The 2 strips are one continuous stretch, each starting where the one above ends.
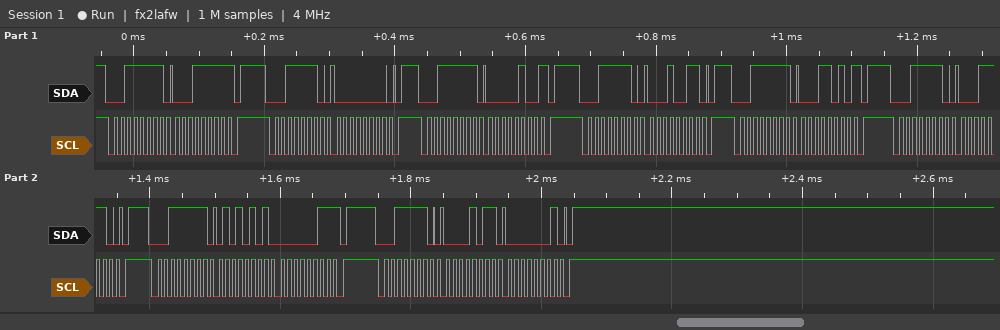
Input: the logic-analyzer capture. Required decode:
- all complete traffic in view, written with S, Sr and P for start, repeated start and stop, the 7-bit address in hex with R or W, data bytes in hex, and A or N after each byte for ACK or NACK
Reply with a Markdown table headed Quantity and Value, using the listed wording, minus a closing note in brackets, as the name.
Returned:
| Quantity | Value |
|---|---|
| all complete traffic in view, written with S, Sr and P for start, repeated start and stop, the 7-bit address in hex with R or W, data bytes in hex, and A or N after each byte for ACK or NACK | S 1FR A 1F N P S 1FW A 00 A P S 1FR A 04 N P S 1FW A 13 A P S 1FR A 1A N P S 1FW A 1E A P S 1FR A 55 A 03 N P S 1FW A 0B A 01 A P |
